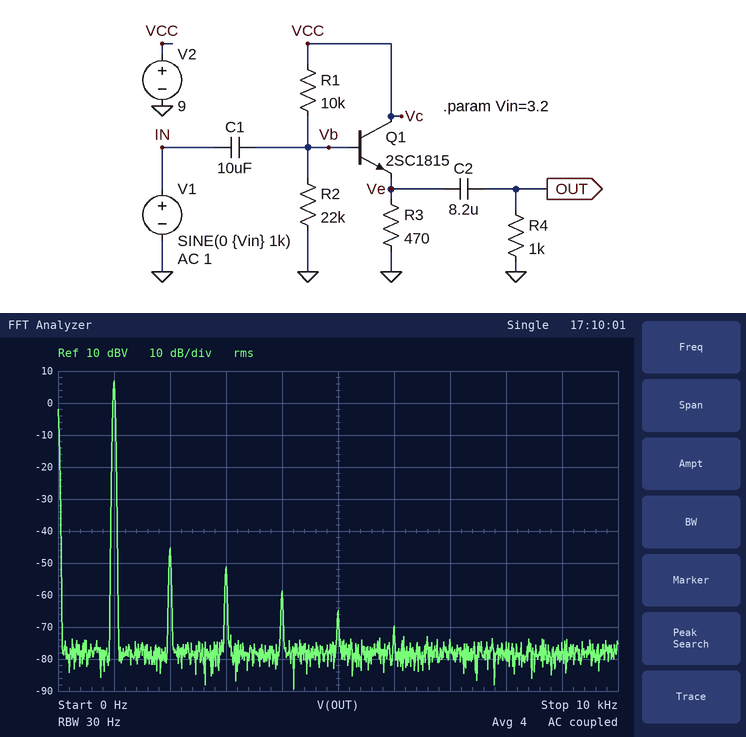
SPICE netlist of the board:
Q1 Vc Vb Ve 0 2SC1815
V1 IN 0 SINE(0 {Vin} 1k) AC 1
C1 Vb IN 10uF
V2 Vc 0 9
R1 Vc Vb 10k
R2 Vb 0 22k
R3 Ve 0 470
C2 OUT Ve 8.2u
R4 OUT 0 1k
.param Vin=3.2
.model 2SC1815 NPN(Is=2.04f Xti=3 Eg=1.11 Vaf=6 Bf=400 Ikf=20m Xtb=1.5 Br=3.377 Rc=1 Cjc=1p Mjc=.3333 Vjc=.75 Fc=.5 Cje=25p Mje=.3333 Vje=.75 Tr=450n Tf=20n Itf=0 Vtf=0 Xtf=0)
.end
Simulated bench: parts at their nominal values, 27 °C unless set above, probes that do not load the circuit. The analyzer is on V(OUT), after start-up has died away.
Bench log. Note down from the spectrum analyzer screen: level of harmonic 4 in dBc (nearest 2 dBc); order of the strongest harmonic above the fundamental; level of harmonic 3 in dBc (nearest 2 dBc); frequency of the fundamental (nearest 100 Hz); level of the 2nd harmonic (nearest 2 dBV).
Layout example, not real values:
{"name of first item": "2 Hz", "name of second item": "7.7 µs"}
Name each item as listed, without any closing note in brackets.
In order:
{"level of harmonic 4 in dBc": "-66 dBc", "order of the strongest harmonic above the fundamental": "2", "level of harmonic 3 in dBc": "-58 dBc", "frequency of the fundamental": "1.0 kHz", "level of the 2nd harmonic": "-46 dBV"}
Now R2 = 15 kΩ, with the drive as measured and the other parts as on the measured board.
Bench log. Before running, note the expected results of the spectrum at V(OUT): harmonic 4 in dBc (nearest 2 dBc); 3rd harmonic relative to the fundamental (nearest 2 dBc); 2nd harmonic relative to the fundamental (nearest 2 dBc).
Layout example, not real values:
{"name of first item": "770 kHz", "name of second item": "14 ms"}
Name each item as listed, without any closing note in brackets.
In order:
{"harmonic 4 in dBc": "-50 dBc", "3rd harmonic relative to the fundamental": "-46 dBc", "2nd harmonic relative to the fundamental": "-42 dBc"}
